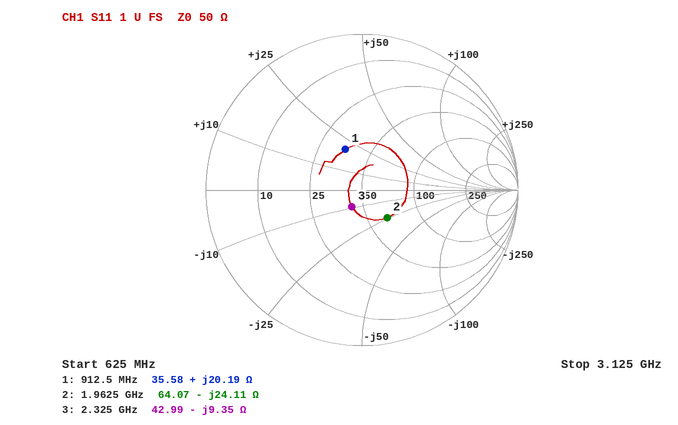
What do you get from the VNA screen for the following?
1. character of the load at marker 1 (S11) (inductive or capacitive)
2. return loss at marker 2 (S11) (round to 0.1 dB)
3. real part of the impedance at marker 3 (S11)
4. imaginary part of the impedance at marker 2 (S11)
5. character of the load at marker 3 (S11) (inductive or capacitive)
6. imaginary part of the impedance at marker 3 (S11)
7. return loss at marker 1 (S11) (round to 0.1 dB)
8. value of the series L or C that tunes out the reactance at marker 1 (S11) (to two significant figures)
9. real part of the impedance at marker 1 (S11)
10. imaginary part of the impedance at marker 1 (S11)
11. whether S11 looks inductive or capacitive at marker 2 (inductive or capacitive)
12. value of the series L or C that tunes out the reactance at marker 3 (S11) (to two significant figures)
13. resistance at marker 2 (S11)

inductive
12.4 dB
42.99 Ω
-24.11 Ω
capacitive
-9.35 Ω
11.0 dB
8.6 pF
35.58 Ω
+20.19 Ω
capacitive
640 pH
64.07 Ω
